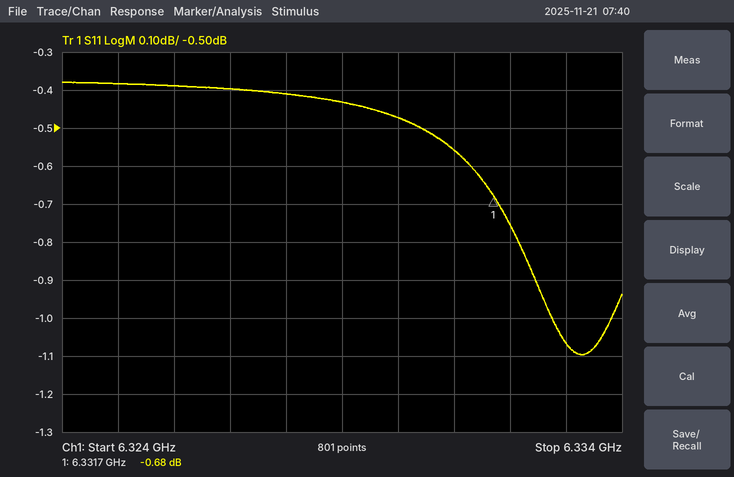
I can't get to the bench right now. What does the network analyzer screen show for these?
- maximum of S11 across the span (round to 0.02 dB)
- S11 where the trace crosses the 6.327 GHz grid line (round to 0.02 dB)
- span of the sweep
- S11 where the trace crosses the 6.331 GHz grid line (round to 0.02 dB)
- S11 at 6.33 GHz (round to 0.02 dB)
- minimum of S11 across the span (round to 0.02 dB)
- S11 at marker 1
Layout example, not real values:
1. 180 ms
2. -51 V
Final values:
1. -0.38 dB
2. -0.40 dB
3. 10 MHz
4. -0.56 dB
5. -0.48 dB
6. -1.10 dB
7. -0.68 dB
